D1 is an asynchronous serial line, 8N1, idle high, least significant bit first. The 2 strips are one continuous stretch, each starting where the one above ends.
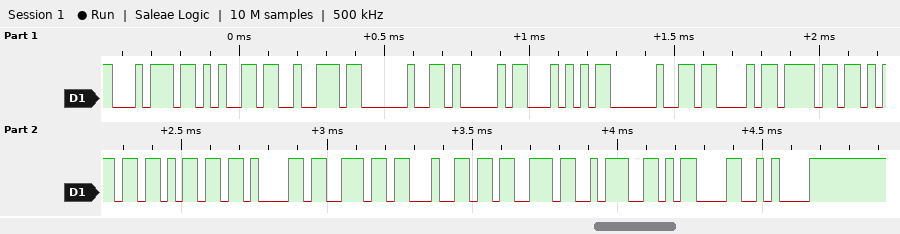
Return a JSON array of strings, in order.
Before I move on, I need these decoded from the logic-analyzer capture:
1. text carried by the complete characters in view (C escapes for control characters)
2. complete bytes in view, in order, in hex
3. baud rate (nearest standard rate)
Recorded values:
["\"ter AT Commands:\\r\\n\"", "74 65 72 20 41 54 20 43 6F 6D 6D 61 6E 64 73 3A 0D 0A", "38400 baud"]
